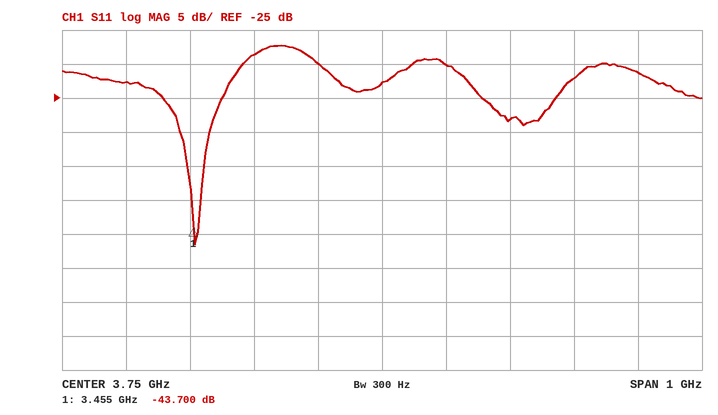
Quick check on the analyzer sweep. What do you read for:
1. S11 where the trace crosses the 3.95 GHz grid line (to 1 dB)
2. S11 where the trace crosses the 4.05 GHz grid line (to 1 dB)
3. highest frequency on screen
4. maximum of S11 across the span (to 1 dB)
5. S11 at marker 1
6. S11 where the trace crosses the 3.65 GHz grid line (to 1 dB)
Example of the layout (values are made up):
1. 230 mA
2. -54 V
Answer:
1. -28 dB
2. -22 dB
3. 4.25 GHz
4. -17 dB
5. -43.700 dB
6. -20 dB
